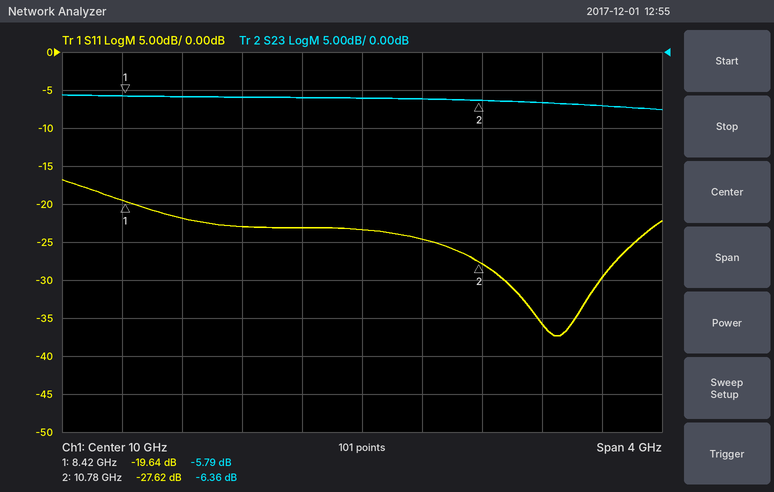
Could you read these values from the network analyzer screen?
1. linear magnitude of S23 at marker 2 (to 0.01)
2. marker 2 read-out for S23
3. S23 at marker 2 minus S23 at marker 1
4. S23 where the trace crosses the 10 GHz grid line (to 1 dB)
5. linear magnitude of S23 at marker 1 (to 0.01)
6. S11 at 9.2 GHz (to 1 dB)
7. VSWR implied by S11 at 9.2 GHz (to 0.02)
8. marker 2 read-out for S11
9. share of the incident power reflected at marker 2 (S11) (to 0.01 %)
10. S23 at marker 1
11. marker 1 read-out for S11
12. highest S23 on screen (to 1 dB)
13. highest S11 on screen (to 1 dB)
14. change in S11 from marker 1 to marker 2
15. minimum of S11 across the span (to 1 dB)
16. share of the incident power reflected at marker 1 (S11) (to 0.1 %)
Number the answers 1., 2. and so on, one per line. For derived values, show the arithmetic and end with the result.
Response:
1. 10^(-6.36/20) ≈ 0.48
2. -6.36 dB
3. -6.36 − (-5.79) = -0.57 dB
4. -6 dB
5. 10^(-5.79/20) ≈ 0.51
6. -23 dB
7. |Γ| = 10^(-23/20) = 0.0708; VSWR = (1 + 0.0708)/(1 − 0.0708) ≈ 1.15, so 1.16 to the nearest 0.02
8. -27.62 dB
9. 10^(-27.62/10) ≈ 0.17 %
10. -5.79 dB
11. -19.64 dB
12. -6 dB
13. -17 dB
14. -27.62 − (-19.64) = -7.98 dB
15. -37 dB
16. 10^(-19.64/10) ≈ 1.1 %
